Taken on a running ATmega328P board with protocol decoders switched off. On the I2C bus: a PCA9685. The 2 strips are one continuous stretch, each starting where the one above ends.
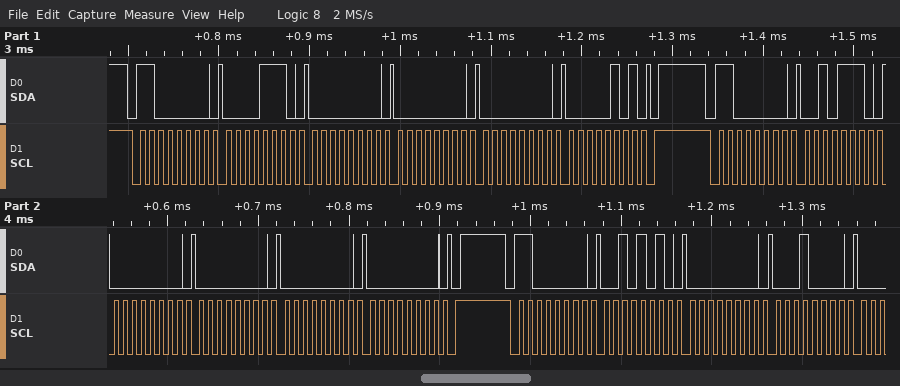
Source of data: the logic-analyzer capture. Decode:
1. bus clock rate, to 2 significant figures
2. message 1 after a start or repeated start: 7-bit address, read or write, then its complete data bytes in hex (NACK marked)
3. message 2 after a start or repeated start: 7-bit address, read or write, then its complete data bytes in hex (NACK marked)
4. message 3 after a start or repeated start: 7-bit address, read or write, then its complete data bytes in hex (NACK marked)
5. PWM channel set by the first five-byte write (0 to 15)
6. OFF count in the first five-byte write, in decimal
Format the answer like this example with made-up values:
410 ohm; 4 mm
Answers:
100 kHz; 0x60 write: 0E 00 00 00 05; 0x60 write: 2E 00 00 00 00; 0x60 write: 2A 00 10; 2; 1280
